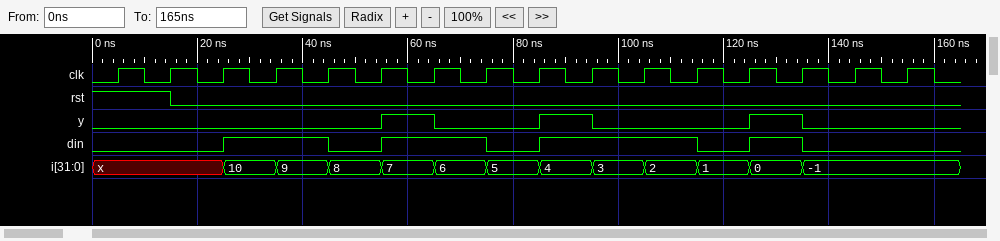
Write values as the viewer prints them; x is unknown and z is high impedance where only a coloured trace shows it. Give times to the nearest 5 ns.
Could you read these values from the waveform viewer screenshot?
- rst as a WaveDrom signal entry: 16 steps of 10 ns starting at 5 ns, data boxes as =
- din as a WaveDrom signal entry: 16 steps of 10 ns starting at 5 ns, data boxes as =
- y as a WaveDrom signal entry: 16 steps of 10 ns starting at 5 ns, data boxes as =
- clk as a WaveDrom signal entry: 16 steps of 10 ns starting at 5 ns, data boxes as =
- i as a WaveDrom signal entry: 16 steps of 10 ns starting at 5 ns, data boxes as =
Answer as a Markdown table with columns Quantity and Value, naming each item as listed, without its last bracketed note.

| Quantity | Value |
|---|---|
| rst as a WaveDrom signal entry: 16 steps of 10 ns starting at 5 ns, data boxes as = | {name: 'rst', wave: '10..............'} |
| din as a WaveDrom signal entry: 16 steps of 10 ns starting at 5 ns, data boxes as = | {name: 'din', wave: '0.1.01.01..010..'} |
| y as a WaveDrom signal entry: 16 steps of 10 ns starting at 5 ns, data boxes as = | {name: 'y', wave: '0....10.10..10..'} |
| clk as a WaveDrom signal entry: 16 steps of 10 ns starting at 5 ns, data boxes as = | {name: 'clk', wave: 'p...............'} |
| i as a WaveDrom signal entry: 16 steps of 10 ns starting at 5 ns, data boxes as = | {name: 'i', wave: 'x.============..', data: '10 9 8 7 6 5 4 3 2 1 0 -1'} |
